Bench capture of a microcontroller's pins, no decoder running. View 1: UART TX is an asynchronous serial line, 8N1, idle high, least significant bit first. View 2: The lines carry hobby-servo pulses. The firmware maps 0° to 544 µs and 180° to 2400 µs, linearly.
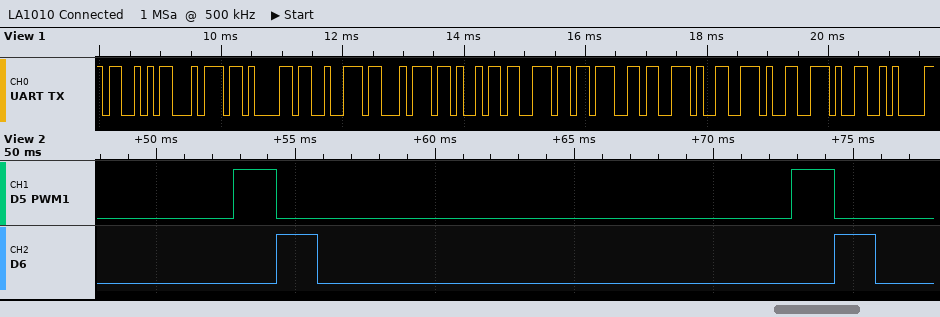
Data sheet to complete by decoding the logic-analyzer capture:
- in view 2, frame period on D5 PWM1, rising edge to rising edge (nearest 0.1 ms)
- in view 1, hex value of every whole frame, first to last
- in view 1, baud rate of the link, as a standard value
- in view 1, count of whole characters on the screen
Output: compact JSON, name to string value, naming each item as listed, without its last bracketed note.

{"in view 2, frame period on D5 PWM1, rising edge to rising edge": "20.0 ms", "in view 1, hex value of every whole frame, first to last": "53 74 61 72 74 69 6E 67 2E 2E 2E 0A", "in view 1, baud rate of the link, as a standard value": "9600 baud", "in view 1, count of whole characters on the screen": "12"}
